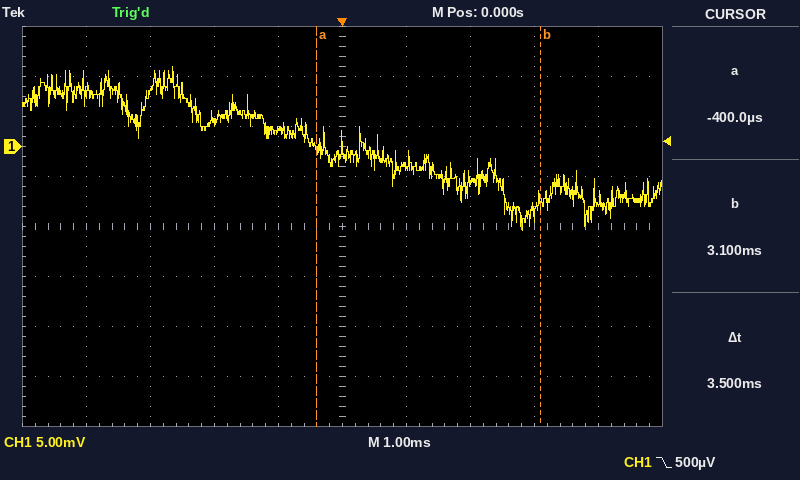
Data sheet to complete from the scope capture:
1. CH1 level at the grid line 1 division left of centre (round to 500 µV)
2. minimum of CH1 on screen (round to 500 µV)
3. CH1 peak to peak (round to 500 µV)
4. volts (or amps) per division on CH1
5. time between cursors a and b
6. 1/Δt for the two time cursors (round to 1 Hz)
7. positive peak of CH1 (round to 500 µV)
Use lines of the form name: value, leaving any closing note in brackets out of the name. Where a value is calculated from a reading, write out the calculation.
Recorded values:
CH1 level at the grid line 1 division left of centre: 1.5 mV
minimum of CH1 on screen: -8.5 mV
CH1 peak to peak: 8.0 mV − (-8.5 mV) = 16.5 mV
volts (or amps) per division on CH1: 5 mV
time between cursors a and b: 3.5 ms
1/Δt for the two time cursors: 1 / 3.5 ms ≈ 286 Hz
positive peak of CH1: 8.0 mV
